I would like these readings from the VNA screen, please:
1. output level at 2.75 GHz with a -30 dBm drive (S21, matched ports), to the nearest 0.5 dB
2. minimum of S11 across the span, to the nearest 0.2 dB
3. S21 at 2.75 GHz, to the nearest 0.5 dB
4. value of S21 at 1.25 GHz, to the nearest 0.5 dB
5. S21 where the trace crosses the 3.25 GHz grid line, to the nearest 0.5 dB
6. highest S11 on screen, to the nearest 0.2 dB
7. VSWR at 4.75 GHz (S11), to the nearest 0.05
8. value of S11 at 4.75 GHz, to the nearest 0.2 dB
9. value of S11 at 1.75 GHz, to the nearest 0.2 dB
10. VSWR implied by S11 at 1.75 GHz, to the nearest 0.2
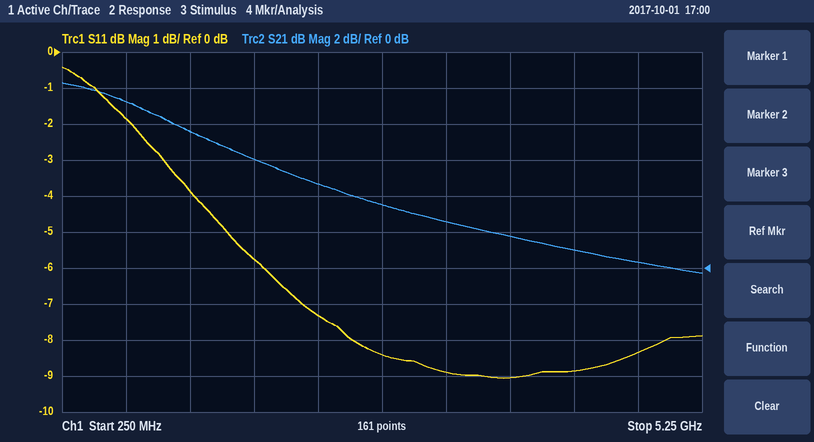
-26.5 dBm
-9.0 dB
3.5 dB
7.5 dB
2.5 dB
-0.4 dB
2.25
-8.4 dB
-5.8 dB
3.2
